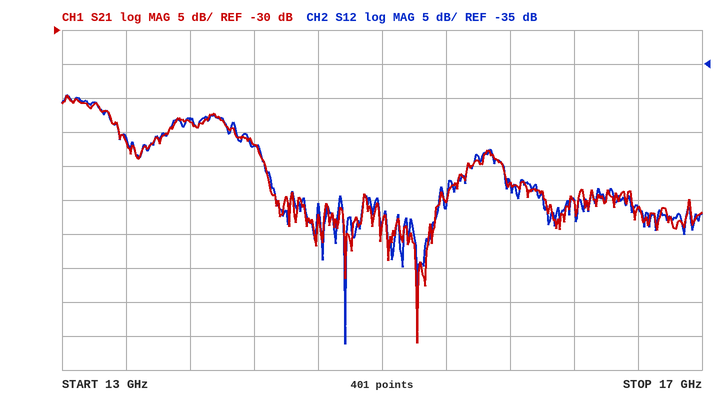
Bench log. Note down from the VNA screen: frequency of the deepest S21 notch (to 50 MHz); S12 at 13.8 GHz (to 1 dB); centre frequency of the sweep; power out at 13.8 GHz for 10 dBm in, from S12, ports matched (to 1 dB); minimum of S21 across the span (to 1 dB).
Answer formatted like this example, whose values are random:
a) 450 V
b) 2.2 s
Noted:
a) 15.20 GHz
b) -43 dB
c) 15 GHz
d) -33 dBm
e) -76 dB
